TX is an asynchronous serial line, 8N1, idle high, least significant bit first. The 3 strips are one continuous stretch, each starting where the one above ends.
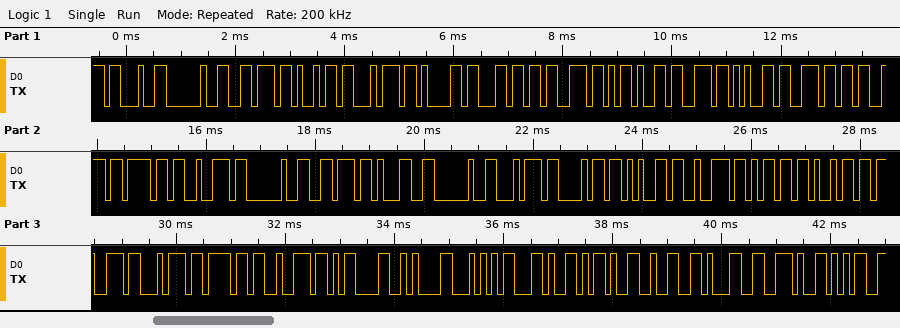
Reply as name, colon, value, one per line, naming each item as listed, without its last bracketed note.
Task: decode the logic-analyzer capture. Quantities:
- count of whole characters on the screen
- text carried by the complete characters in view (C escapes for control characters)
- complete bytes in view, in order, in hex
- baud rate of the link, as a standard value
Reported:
count of whole characters on the screen: 38
text carried by the complete characters in view: "# vitals-sensor v1 thermistor\r\nT,-21.5"
complete bytes in view, in order, in hex: 23 20 76 69 74 61 6C 73 2D 73 65 6E 73 6F 72 20 76 31 20 74 68 65 72 6D 69 73 74 6F 72 0D 0A 54 2C 2D 32 31 2E 35
baud rate of the link, as a standard value: 9600 baud
